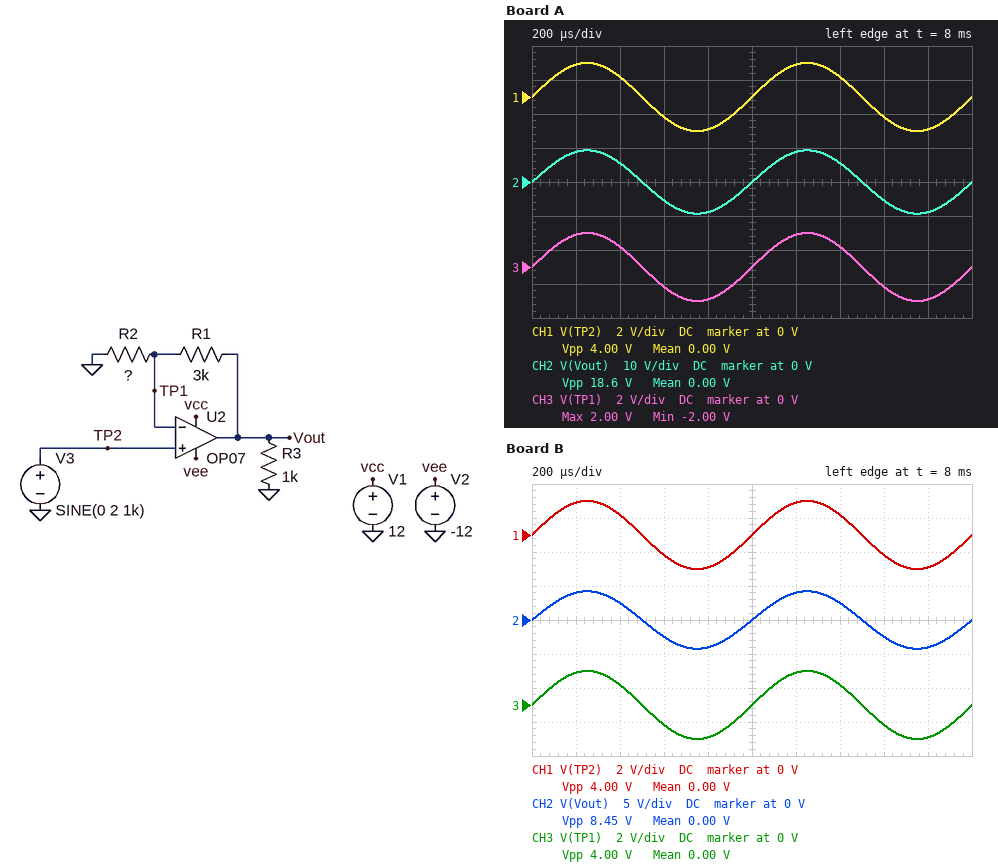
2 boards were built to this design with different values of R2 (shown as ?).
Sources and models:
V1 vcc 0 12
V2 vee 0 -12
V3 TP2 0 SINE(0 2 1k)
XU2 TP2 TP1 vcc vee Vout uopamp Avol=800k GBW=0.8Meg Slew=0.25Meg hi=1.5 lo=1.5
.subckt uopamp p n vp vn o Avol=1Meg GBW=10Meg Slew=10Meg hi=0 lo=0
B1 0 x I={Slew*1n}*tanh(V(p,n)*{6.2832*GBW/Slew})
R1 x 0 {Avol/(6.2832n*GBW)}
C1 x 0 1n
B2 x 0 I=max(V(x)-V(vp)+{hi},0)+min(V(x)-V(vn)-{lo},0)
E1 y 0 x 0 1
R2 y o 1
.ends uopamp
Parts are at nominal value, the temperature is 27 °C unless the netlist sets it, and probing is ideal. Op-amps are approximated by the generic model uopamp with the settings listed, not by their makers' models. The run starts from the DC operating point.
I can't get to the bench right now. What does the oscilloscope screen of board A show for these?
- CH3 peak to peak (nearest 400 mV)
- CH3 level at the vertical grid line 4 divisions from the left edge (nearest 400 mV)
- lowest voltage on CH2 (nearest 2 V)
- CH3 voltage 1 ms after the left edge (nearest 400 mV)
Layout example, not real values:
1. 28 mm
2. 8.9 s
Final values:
1. 4.0 V
2. -2.0 V
3. -10 V
4. 0 V
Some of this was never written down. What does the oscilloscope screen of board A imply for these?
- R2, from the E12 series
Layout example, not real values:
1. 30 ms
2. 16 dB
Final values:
1. 820 Ω
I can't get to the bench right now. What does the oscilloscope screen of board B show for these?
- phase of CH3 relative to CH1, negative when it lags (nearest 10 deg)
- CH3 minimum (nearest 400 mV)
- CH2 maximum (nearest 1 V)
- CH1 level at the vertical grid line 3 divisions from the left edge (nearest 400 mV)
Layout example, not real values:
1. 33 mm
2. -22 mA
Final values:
1. 0 deg
2. -2.0 V
3. 4 V
4. -1.2 V
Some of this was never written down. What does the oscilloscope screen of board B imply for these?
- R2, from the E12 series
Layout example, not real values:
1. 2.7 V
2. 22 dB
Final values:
1. 2.7 kΩ
